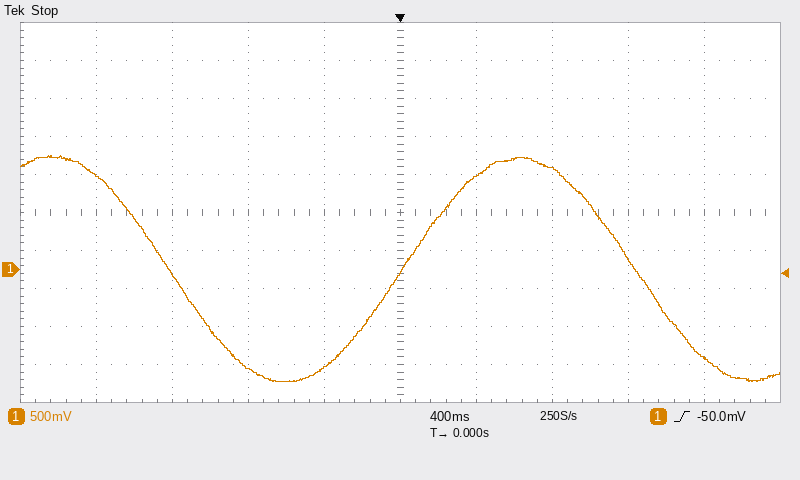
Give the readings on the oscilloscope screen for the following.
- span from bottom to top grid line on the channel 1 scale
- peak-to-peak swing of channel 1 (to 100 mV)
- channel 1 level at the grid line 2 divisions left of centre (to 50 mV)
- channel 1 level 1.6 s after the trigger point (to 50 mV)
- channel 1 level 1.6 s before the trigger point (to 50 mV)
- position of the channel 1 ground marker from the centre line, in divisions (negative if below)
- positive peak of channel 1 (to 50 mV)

5 V
3.00 V
-1.30 V
-1.15 V
1.25 V
-1.5 div
1.50 V
